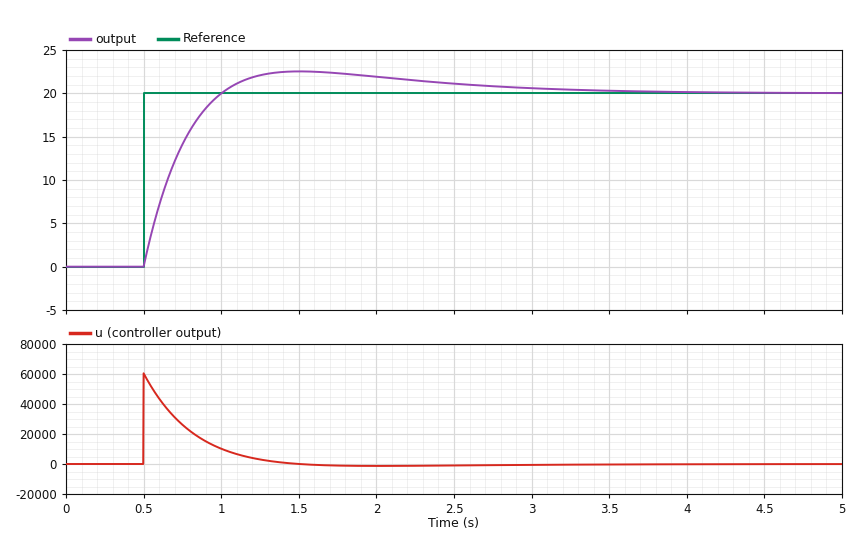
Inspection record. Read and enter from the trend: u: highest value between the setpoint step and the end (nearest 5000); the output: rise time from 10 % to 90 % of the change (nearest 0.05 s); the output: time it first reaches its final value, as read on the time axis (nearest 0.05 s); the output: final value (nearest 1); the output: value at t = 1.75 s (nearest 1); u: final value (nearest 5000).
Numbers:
60000
0.35 s
1.00 s
20
22
0
